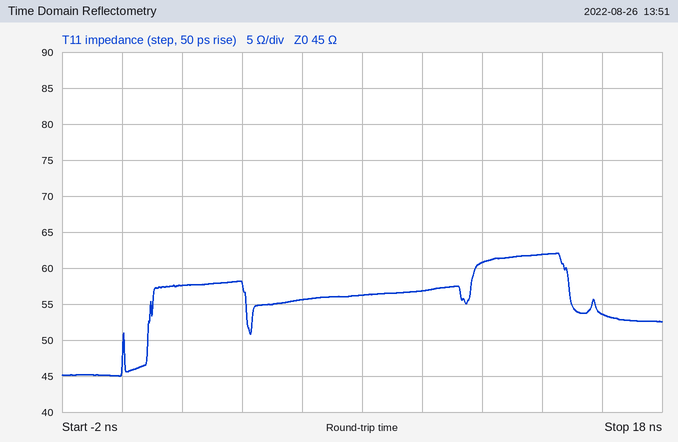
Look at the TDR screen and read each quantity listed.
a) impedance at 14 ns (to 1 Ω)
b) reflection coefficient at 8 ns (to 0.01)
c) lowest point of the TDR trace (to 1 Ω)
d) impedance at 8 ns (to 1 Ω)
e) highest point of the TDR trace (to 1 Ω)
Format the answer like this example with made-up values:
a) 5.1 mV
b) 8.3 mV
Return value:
a) 62 Ω
b) +0.11
c) 45 Ω
d) 56 Ω
e) 62 Ω
